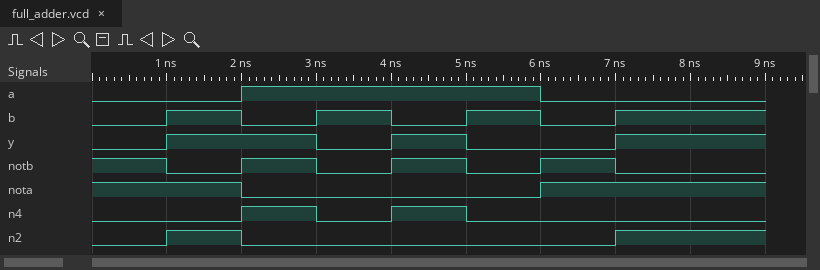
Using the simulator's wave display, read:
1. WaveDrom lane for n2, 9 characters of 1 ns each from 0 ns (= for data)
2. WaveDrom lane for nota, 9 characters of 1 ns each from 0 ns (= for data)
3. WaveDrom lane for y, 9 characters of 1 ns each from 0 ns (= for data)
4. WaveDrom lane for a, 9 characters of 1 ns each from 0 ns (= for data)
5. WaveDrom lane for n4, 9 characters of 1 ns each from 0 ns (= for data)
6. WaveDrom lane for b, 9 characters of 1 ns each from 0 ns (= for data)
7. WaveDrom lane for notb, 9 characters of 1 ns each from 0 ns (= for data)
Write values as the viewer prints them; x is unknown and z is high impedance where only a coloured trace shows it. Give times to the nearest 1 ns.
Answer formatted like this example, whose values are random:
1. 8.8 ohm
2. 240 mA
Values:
1. {name: 'n2', wave: '010....1.'}
2. {name: 'nota', wave: '1.0...1..'}
3. {name: 'y', wave: '01.010.1.'}
4. {name: 'a', wave: '0.1...0..'}
5. {name: 'n4', wave: '0.1010...'}
6. {name: 'b', wave: '01010101.'}
7. {name: 'notb', wave: '10101010.'}
